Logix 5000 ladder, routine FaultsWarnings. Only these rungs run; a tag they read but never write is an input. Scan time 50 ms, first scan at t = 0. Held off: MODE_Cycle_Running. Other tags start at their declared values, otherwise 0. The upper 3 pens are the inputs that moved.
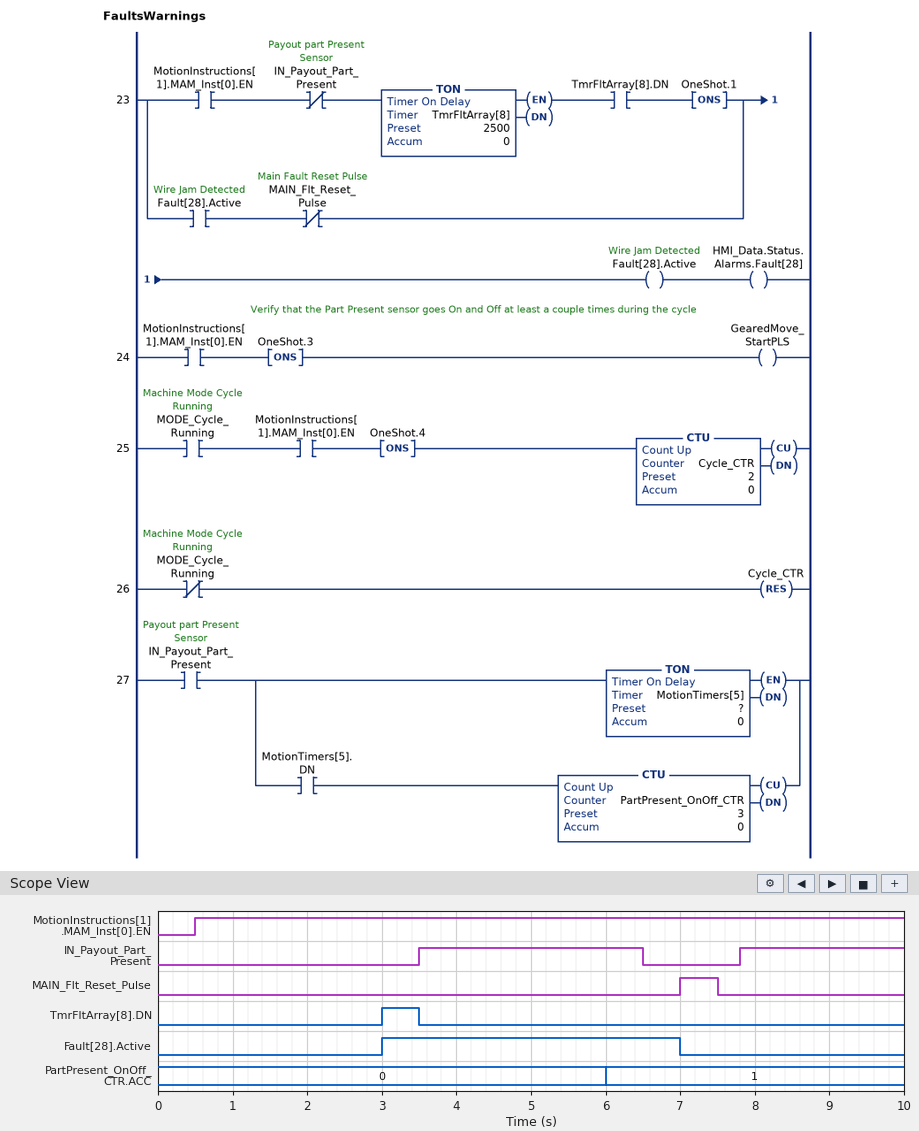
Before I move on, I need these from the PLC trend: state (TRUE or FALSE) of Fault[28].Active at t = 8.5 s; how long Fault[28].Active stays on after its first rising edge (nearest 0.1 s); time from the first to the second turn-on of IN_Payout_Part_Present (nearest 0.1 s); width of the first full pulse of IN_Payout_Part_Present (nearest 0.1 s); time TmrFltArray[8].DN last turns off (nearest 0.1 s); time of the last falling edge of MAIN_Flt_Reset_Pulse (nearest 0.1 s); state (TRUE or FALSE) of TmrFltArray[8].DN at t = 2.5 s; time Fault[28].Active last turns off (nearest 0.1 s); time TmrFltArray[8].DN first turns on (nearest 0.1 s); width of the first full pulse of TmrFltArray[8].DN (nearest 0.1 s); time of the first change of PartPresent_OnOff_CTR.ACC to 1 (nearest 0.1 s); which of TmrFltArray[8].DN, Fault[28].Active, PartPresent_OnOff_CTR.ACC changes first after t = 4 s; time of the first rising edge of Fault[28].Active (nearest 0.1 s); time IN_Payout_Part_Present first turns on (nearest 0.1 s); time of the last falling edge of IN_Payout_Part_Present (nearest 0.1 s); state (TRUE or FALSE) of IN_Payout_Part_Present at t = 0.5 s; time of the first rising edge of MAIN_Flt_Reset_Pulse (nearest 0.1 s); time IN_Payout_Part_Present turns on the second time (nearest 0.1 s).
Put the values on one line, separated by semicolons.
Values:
FALSE; 4.0 s; 4.3 s; 3.0 s; 3.5 s; 7.5 s; FALSE; 7.0 s; 3.0 s; 0.5 s; 6.0 s; PartPresent_OnOff_CTR.ACC; 3.0 s; 3.5 s; 6.5 s; FALSE; 7.0 s; 7.8 s
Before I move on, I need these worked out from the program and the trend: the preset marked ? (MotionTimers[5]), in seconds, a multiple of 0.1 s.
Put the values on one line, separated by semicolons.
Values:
2.5 s
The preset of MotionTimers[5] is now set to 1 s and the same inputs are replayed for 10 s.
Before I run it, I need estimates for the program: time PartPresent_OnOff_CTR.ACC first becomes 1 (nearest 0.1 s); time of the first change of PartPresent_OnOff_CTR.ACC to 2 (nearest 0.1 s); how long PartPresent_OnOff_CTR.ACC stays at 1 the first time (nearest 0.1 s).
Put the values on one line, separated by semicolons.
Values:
4.5 s; 8.8 s; 4.3 s
